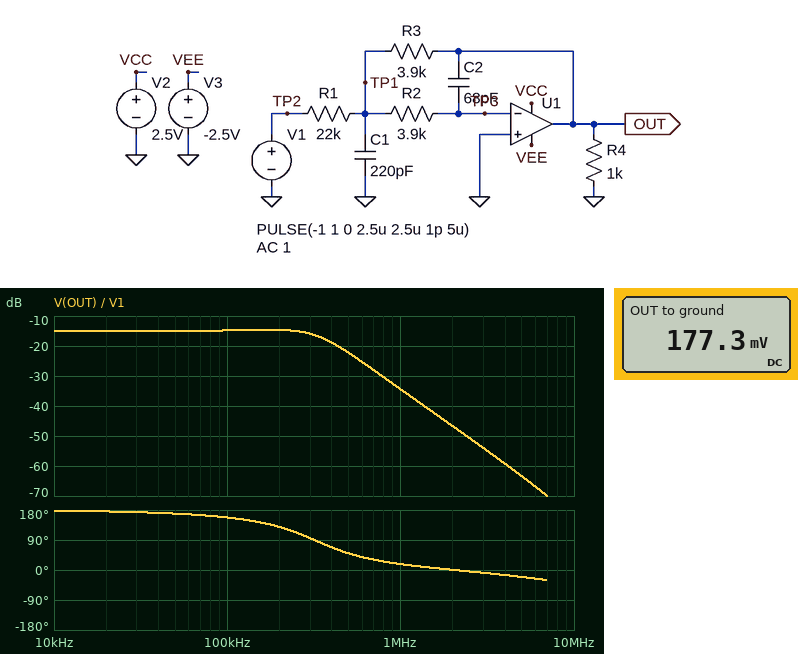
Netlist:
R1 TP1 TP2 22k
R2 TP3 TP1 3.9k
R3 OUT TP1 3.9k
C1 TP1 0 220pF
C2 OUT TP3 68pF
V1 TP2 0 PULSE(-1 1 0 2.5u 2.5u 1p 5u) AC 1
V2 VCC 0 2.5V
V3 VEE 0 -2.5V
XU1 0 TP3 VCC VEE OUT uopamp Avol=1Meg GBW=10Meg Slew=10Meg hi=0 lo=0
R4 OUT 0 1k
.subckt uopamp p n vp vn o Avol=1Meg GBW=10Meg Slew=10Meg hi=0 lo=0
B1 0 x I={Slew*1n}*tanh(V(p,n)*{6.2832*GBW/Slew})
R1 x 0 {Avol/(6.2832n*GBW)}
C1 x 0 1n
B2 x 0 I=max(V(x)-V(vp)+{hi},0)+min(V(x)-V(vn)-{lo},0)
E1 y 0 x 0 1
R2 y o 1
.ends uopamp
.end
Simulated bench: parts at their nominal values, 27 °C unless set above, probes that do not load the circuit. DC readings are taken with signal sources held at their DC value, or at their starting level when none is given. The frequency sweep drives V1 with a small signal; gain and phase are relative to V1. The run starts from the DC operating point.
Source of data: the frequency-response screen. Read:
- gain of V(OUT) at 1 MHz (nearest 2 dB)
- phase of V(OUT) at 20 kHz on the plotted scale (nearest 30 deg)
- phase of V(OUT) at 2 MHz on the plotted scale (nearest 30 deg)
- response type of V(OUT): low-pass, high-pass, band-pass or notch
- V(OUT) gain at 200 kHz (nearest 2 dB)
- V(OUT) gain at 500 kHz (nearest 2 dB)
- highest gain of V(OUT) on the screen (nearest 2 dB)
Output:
-34 dB
180 deg
0 deg
low-pass
-14 dB
-22 dB
-14 dB
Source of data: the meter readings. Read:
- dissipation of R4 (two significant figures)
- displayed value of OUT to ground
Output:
31 µW
177.3 mV
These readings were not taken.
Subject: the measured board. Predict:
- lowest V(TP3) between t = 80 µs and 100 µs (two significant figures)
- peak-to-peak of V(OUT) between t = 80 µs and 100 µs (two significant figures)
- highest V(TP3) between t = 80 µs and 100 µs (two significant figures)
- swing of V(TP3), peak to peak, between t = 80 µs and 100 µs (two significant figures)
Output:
-2.7 mV
310 mV
2.7 mV
5.5 mV
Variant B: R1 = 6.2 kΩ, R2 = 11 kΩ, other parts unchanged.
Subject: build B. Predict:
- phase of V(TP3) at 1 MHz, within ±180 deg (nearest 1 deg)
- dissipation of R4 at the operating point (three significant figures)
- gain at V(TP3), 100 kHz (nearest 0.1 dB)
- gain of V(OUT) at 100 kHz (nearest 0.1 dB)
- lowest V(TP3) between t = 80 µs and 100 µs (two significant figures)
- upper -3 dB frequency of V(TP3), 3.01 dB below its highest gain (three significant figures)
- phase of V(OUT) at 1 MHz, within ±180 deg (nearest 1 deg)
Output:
-75 deg
396 µW
-45.6 dB
-5.6 dB
-5.8 mV
448 kHz
15 deg
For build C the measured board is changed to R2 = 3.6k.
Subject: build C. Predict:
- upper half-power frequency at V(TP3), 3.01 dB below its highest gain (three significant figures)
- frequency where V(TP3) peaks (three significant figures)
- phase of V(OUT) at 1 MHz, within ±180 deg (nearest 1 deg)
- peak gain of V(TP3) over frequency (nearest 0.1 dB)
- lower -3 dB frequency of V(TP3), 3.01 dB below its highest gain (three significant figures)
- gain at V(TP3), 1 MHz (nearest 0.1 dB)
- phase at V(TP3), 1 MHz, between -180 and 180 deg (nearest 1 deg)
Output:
587 kHz
336 kHz
19 deg
-45.9 dB
192 kHz
-53.7 dB
-71 deg
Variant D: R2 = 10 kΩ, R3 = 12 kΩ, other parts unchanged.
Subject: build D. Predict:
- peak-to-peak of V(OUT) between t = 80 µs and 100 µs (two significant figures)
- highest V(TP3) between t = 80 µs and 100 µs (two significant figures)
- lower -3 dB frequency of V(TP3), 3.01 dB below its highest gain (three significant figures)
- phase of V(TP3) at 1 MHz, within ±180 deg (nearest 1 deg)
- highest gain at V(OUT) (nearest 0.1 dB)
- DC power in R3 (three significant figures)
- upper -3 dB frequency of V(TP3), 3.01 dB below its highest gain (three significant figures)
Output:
290 mV
3.0 mV
61.5 kHz
-86 deg
-5.3 dB
24.8 µW
224 kHz
